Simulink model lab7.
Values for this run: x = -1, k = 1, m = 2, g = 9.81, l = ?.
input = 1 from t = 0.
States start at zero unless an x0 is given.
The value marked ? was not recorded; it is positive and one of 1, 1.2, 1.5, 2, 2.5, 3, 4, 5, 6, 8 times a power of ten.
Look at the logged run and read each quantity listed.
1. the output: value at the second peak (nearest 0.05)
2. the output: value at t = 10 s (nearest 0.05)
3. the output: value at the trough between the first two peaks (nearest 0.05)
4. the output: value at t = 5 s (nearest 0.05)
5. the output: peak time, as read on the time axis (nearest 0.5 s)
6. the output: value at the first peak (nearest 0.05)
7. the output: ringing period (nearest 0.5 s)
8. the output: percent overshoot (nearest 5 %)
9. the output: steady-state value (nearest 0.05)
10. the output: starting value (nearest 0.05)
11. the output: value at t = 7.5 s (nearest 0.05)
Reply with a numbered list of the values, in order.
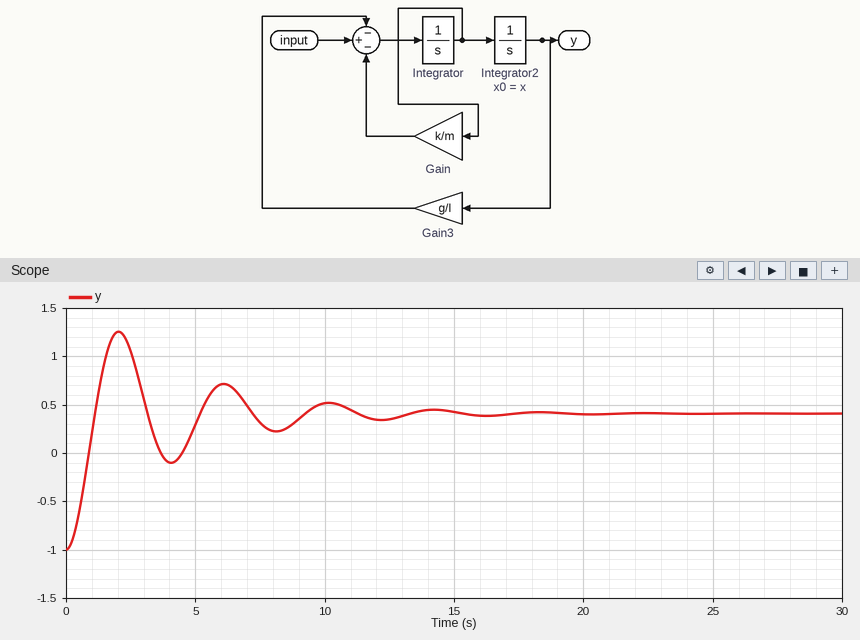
1. 0.70
2. 0.50
3. -0.10
4. 0.30
5. 2.0 s
6. 1.25
7. 4.0 s
8. 60 %
9. 0.40
10. -1.00
11. 0.30
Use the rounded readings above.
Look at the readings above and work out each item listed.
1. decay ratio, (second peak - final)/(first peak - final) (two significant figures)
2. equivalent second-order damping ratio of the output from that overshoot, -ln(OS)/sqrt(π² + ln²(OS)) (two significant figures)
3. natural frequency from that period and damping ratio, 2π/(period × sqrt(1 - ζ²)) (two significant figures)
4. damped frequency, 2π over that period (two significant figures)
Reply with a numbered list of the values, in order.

1. 0.35
2. 0.16
3. 1.6 rad/s
4. 1.6 rad/s
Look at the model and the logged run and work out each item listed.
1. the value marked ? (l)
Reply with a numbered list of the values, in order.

1. 4
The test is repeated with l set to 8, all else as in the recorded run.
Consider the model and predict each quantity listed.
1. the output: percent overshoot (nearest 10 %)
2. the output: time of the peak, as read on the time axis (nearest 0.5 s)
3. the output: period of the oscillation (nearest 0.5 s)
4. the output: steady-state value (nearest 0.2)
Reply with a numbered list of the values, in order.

1. 50 %
2. 3.0 s
3. 6.0 s
4. 0.8
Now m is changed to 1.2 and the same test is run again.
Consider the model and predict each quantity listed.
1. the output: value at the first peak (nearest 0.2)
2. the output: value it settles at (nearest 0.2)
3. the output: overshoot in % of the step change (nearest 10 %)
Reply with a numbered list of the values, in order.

1. 1.0
2. 0.4
3. 40 %
